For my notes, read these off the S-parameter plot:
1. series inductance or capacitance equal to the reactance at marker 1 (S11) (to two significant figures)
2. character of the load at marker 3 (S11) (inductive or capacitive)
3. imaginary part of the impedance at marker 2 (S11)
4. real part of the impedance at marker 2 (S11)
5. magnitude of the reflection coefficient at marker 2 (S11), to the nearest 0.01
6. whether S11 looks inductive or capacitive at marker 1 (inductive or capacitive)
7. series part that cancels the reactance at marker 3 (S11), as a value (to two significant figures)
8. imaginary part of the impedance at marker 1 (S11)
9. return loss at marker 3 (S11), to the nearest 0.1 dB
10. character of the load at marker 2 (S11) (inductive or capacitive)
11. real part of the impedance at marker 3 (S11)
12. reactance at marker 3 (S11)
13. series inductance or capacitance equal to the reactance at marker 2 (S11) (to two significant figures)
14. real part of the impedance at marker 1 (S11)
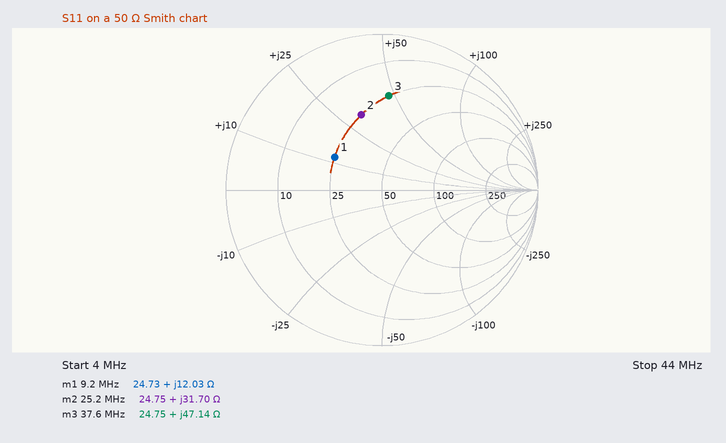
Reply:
210 nH
inductive
+31.70 Ω
24.75 Ω
0.50
inductive
90 pF
+12.03 Ω
4.4 dB
inductive
24.75 Ω
+47.14 Ω
200 nH
24.73 Ω
